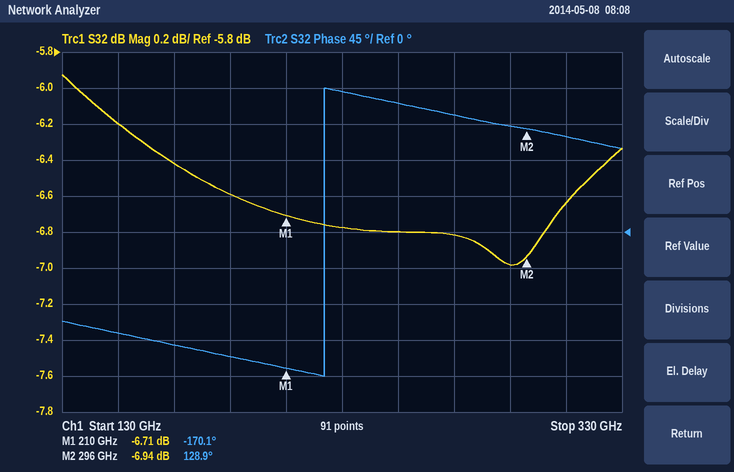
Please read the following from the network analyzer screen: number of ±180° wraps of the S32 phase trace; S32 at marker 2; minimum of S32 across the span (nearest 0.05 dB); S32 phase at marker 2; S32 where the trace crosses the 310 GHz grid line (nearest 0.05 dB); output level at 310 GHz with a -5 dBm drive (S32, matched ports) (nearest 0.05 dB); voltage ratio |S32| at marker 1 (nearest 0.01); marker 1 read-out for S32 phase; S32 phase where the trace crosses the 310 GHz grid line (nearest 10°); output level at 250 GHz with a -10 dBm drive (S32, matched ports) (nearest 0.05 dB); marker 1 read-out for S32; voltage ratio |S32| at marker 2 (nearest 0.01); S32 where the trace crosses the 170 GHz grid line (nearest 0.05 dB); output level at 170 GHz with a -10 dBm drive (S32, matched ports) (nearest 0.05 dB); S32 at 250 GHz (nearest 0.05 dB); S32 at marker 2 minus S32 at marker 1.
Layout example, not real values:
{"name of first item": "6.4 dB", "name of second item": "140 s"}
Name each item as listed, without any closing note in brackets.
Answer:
{"number of ±180° wraps of the S32 phase trace": "1", "S32 at marker 2": "-6.94 dB", "minimum of S32 across the span": "-7.00 dB", "S32 phase at marker 2": "128.9°", "S32 where the trace crosses the 310 GHz grid line": "-6.65 dB", "output level at 310 GHz with a -5 dBm drive (S32, matched ports)": "-11.65 dBm", "voltage ratio |S32| at marker 1": "0.46", "marker 1 read-out for S32 phase": "-170.1°", "S32 phase where the trace crosses the 310 GHz grid line": "120°", "output level at 250 GHz with a -10 dBm drive (S32, matched ports)": "-16.80 dBm", "marker 1 read-out for S32": "-6.71 dB", "voltage ratio |S32| at marker 2": "0.45", "S32 where the trace crosses the 170 GHz grid line": "-6.40 dB", "output level at 170 GHz with a -10 dBm drive (S32, matched ports)": "-16.40 dBm", "S32 at 250 GHz": "-6.80 dB", "S32 at marker 2 minus S32 at marker 1": "-0.23 dB"}
